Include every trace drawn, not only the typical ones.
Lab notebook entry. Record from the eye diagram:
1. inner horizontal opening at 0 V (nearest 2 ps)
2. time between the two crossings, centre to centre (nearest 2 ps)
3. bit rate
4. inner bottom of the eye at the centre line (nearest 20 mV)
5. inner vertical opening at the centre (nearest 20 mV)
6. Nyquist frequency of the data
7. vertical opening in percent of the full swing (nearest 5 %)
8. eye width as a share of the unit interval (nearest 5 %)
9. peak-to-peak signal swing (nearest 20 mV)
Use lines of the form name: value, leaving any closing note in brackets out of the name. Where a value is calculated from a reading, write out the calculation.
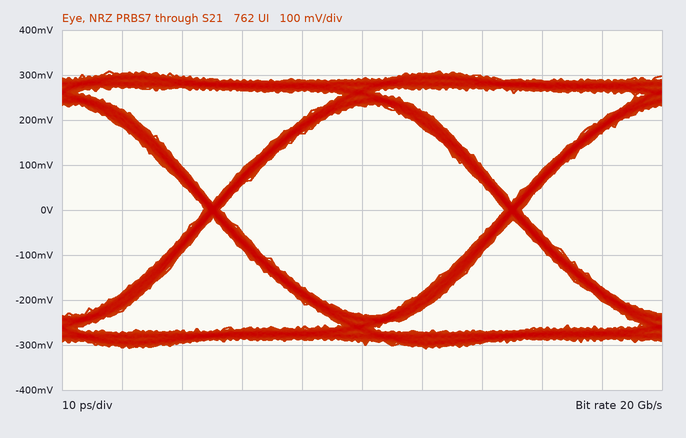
inner horizontal opening at 0 V: 48 ps
time between the two crossings, centre to centre: 50 ps
bit rate: 20 Gb/s
inner bottom of the eye at the centre line: -240 mV
inner vertical opening at the centre: 460 mV
Nyquist frequency of the data: 10 GHz
vertical opening in percent of the full swing: 460 mV / 620 mV ≈ 74.2 %, so 75 % to the nearest 5 %
eye width as a share of the unit interval: 48 ps / 50 ps ≈ 96.0 %, so 95 % to the nearest 5 %
peak-to-peak signal swing: 620 mV
